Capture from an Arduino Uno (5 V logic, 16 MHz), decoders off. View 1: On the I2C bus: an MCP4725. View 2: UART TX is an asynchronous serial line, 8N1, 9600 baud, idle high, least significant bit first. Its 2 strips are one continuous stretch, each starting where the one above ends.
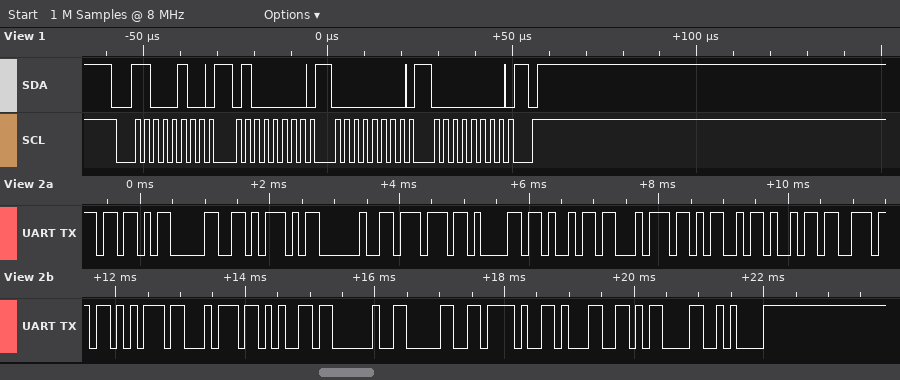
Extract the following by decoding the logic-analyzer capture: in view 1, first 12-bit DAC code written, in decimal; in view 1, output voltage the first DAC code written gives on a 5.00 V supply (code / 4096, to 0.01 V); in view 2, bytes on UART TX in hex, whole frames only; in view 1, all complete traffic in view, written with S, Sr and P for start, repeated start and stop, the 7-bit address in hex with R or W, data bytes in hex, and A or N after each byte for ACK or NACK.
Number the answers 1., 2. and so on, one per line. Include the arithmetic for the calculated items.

1. 0
2. 0 / 4096 x 5.00 V = 0.00 V
3. 5B 30 5D 20 77 61 69 74 4D 69 6E 75 74 65 20 30 2F 31 0D 0A
4. S 62W A 40 A 00 A 00 A P
